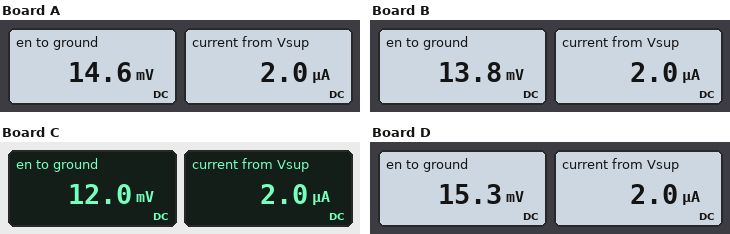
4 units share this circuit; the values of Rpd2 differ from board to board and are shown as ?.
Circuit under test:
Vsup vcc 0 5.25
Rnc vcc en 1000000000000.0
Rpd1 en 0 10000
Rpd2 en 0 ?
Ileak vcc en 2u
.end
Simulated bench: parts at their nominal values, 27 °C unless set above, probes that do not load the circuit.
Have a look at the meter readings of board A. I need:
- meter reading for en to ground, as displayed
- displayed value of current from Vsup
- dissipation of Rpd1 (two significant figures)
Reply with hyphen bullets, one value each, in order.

- 14.6 mV
- 2.0 µA
- 21 nW
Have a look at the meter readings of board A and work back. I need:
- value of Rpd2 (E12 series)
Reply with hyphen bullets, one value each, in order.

- 27 kΩ
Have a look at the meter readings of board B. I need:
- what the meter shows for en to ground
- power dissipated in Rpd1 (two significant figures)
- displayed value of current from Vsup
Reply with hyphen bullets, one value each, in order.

- 13.8 mV
- 19 nW
- 2.0 µA
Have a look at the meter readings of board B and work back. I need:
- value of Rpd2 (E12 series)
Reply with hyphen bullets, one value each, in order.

- 22 kΩ
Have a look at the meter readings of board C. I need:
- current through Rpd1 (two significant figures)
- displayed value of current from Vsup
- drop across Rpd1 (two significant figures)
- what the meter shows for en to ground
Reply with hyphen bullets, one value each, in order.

- 1.2 µA
- 2.0 µA
- 12 mV
- 12.0 mV
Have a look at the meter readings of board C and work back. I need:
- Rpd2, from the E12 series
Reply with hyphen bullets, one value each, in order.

- 15 kΩ
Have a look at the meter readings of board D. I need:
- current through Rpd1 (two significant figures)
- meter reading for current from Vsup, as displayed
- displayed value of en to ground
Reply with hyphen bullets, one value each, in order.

- 1.5 µA
- 2.0 µA
- 15.3 mV
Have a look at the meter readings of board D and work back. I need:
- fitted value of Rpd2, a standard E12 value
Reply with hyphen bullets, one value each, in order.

- 33 kΩ
